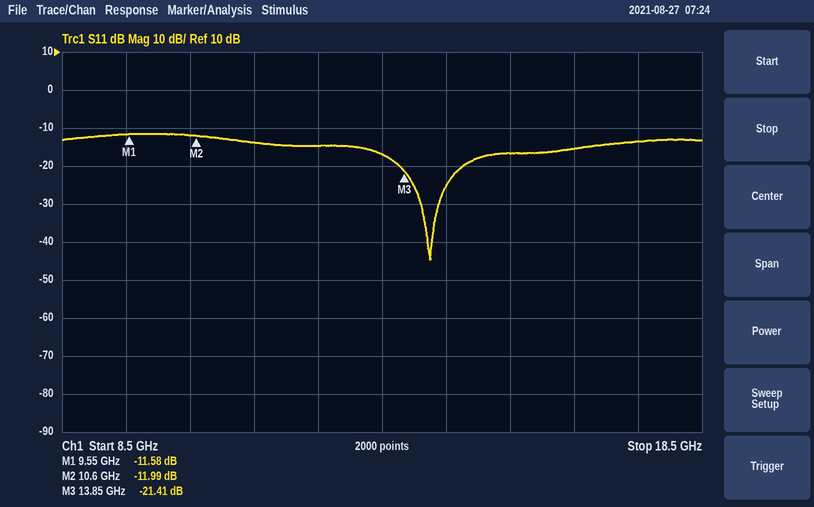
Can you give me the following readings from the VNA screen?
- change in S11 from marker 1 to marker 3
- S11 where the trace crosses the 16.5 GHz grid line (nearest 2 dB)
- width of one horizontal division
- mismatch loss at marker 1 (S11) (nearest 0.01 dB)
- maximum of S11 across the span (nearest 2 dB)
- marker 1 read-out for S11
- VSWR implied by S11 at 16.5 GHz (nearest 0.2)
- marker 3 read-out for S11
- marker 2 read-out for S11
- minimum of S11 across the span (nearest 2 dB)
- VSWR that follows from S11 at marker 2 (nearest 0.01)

-9.83 dB
-16 dB
1 GHz
0.31 dB
-12 dB
-11.58 dB
1.4
-21.41 dB
-11.99 dB
-44 dB
1.67
